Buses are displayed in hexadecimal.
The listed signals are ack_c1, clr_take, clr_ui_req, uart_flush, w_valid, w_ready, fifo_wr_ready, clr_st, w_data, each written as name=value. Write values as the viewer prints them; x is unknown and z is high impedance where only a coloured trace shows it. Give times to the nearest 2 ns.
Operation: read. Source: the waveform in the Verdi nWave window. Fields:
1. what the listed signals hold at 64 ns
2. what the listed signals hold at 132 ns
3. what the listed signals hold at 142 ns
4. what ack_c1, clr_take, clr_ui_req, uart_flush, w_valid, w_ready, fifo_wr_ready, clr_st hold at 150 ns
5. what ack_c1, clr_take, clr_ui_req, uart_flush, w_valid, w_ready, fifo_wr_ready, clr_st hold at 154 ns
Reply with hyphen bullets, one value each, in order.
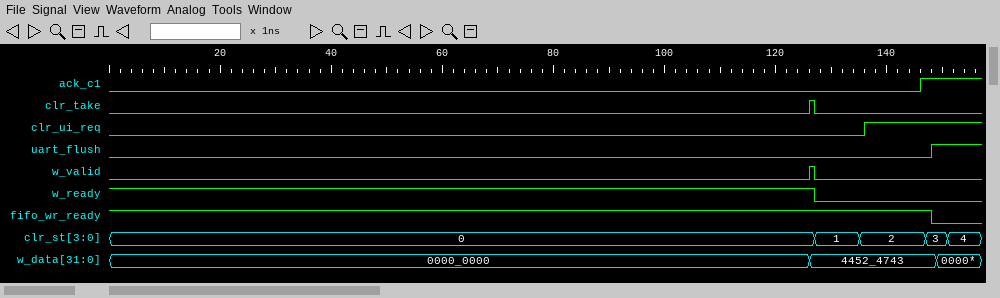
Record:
- ack_c1=0, clr_take=0, clr_ui_req=0, uart_flush=0, w_valid=0, w_ready=1, fifo_wr_ready=1, clr_st=0, w_data=0000_0000
- ack_c1=0, clr_take=0, clr_ui_req=0, uart_flush=0, w_valid=0, w_ready=0, fifo_wr_ready=1, clr_st=1, w_data=4452_4743
- ack_c1=0, clr_take=0, clr_ui_req=1, uart_flush=0, w_valid=0, w_ready=0, fifo_wr_ready=1, clr_st=2, w_data=4452_4743
- ack_c1=1, clr_take=0, clr_ui_req=1, uart_flush=1, w_valid=0, w_ready=0, fifo_wr_ready=0, clr_st=3
- ack_c1=1, clr_take=0, clr_ui_req=1, uart_flush=1, w_valid=0, w_ready=0, fifo_wr_ready=0, clr_st=4
